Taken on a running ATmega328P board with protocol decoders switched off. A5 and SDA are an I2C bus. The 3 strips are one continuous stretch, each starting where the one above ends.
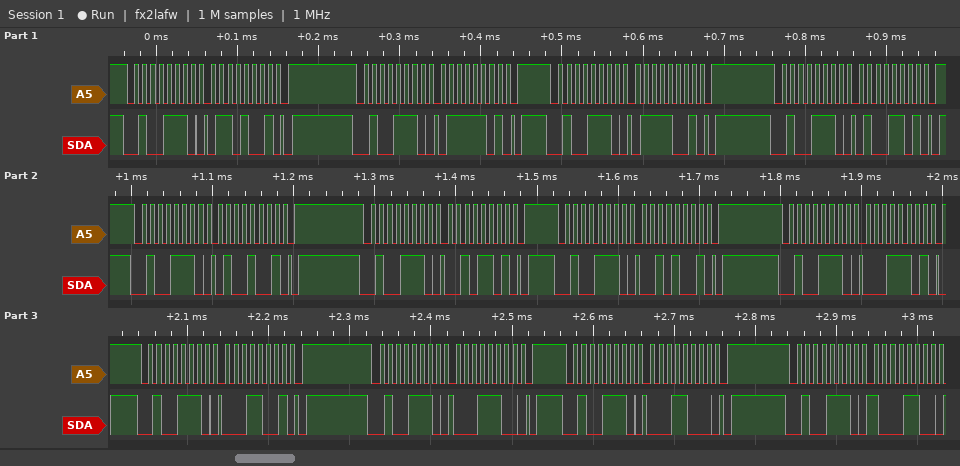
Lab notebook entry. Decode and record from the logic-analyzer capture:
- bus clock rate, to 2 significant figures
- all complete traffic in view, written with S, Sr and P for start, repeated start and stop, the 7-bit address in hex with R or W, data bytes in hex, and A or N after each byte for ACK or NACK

100 kHz
S 27W A 69 A P S 27W A 7D A P S 27W A 79 A P S 27W A 4D A P S 27W A 49 A P S 27W A 2D A P S 27W A 29 A P S 27W A 1D A P S 27W A 19 A P S 27W A 1C A P S 27W A 18 A P S 27W A 8C A
